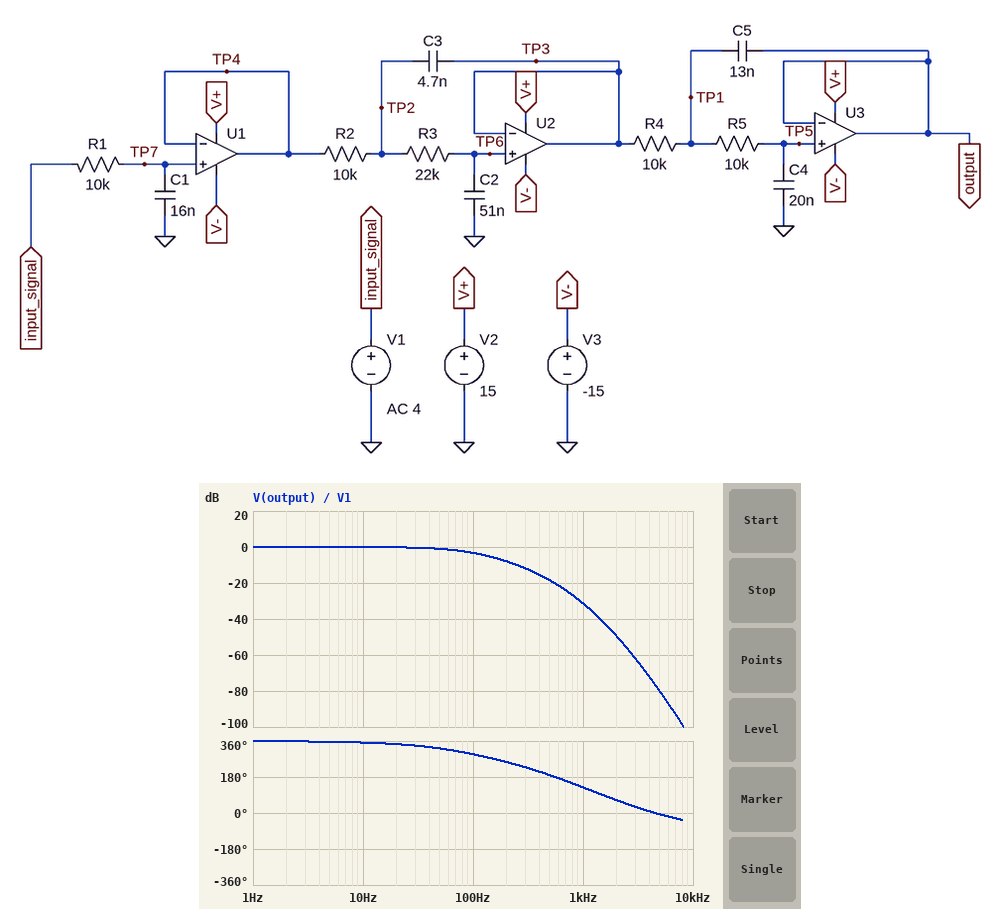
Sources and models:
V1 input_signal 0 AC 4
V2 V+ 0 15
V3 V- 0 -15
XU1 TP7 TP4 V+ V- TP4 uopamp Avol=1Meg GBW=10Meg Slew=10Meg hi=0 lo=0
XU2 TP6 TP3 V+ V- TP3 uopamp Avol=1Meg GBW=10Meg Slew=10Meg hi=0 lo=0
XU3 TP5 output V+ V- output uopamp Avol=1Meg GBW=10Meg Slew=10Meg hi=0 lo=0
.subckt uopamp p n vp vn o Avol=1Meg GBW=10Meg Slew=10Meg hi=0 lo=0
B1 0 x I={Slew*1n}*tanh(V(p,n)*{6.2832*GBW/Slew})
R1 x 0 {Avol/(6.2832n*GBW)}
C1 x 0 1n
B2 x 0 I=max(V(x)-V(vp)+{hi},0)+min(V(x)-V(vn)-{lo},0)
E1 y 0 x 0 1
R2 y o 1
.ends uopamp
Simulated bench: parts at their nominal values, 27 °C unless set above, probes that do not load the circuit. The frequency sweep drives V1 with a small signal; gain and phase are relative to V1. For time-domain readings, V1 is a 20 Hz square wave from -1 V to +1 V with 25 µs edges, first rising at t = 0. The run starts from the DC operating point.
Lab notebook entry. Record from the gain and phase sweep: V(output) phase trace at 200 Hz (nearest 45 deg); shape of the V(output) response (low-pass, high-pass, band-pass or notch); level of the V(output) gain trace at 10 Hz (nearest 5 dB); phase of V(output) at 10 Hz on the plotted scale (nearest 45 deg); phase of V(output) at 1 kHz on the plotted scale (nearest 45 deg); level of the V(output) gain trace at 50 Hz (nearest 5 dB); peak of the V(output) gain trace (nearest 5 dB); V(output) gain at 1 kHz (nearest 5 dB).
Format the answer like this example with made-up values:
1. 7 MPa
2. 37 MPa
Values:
1. 270 deg
2. low-pass
3. 0 dB
4. 360 deg
5. 135 deg
6. 0 dB
7. 0 dB
8. -30 dB
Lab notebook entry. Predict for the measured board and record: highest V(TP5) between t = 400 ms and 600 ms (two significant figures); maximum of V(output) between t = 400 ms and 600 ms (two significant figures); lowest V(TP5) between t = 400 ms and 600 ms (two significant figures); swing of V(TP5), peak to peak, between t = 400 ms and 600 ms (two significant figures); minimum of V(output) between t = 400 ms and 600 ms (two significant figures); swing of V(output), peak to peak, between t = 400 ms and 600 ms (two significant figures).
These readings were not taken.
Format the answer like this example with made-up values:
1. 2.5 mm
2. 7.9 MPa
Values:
1. 1.0 V
2. 1.0 V
3. -1.0 V
4. 2.0 V
5. -1.0 V
6. 2.0 V
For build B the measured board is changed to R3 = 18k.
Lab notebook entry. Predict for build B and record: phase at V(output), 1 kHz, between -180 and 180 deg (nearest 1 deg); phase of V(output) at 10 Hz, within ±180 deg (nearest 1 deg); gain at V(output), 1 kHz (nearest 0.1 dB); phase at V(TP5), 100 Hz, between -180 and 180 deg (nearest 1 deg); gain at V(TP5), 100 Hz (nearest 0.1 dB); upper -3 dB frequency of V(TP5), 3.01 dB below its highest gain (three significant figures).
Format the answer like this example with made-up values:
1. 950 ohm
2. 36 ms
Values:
1. 130 deg
2. -7 deg
3. -30.1 dB
4. -62 deg
5. -2.7 dB
6. 107 Hz
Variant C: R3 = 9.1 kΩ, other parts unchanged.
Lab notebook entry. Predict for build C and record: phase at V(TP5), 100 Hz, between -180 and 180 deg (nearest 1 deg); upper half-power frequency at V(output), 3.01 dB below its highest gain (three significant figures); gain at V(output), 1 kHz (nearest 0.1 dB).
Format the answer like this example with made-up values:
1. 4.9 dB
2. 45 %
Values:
1. -52 deg
2. 148 Hz
3. -26.8 dB
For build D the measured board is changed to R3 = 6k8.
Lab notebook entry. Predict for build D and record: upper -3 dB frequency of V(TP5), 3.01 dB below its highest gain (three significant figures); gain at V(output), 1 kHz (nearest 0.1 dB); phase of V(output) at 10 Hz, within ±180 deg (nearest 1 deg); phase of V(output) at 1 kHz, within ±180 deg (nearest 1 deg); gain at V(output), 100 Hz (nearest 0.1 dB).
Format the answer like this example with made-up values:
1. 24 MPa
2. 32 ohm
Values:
1. 164 Hz
2. -25.7 dB
3. -5 deg
4. 138 deg
5. -1.3 dB
